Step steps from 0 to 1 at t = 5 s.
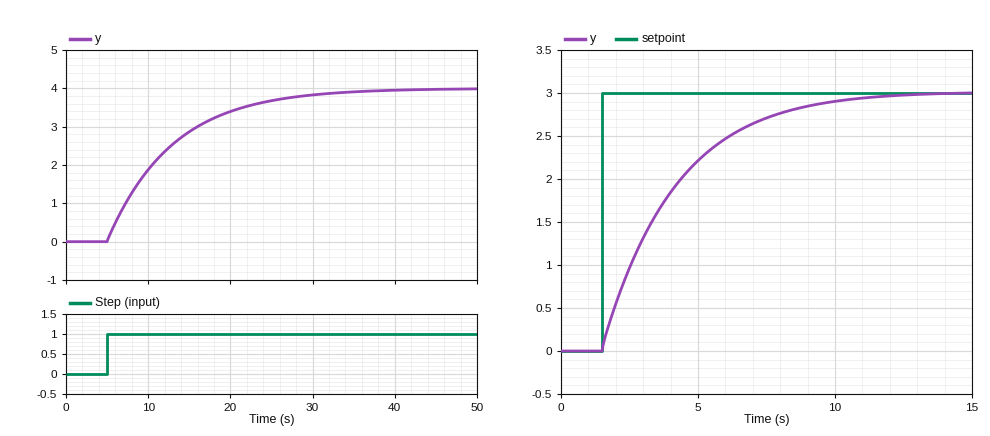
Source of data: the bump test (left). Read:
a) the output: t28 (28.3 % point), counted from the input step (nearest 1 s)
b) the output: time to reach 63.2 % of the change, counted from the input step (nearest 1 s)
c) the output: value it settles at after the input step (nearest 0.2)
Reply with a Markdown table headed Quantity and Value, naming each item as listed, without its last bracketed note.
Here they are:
| Quantity | Value |
|---|---|
| the output: t28 (28.3 % point), counted from the input step | 3 s |
| the output: time to reach 63.2 % of the change, counted from the input step | 8 s |
| the output: value it settles at after the input step | 4.0 |
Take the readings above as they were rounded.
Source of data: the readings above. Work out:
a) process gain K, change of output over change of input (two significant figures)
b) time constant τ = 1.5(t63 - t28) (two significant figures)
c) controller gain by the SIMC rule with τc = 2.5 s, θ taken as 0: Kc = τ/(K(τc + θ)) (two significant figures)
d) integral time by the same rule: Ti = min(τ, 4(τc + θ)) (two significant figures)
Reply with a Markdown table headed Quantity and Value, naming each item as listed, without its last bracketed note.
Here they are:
| Quantity | Value |
|---|---|
| process gain K, change of output over change of input | 4.0 |
| time constant τ = 1.5(t63 - t28) | 7.5 s |
| controller gain by the SIMC rule with τc = 2.5 s, θ taken as 0: Kc = τ/(K(τc + θ)) | 0.75 |
| integral time by the same rule: Ti = min(τ, 4(τc + θ)) | 7.5 s |
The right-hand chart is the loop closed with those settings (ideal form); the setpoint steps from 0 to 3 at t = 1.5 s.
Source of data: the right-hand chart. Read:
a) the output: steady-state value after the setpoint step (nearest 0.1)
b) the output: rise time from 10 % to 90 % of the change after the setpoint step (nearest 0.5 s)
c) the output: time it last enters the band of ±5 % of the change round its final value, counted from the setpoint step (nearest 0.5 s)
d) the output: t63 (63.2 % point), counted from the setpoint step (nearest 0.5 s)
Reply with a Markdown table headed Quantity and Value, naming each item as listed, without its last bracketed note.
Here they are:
| Quantity | Value |
|---|---|
| the output: steady-state value after the setpoint step | 3.0 |
| the output: rise time from 10 % to 90 % of the change after the setpoint step | 5.5 s |
| the output: time it last enters the band of ±5 % of the change round its final value, counted from the setpoint step | 7.5 s |
| the output: t63 (63.2 % point), counted from the setpoint step | 2.5 s |
